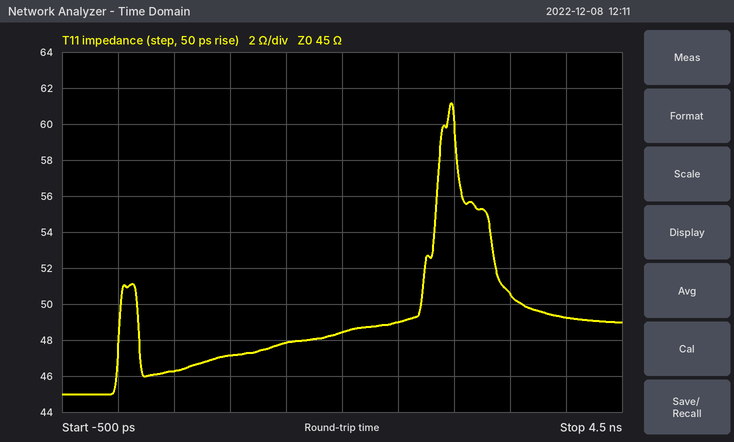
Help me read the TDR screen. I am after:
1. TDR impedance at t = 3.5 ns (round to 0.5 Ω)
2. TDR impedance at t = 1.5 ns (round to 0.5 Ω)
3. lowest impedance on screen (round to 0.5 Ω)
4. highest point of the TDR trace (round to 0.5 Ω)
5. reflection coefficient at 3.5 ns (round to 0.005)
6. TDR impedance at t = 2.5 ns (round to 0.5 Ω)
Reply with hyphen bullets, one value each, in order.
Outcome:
- 50.5 Ω
- 48.0 Ω
- 45.0 Ω
- 61.0 Ω
- +0.060
- 49.0 Ω
